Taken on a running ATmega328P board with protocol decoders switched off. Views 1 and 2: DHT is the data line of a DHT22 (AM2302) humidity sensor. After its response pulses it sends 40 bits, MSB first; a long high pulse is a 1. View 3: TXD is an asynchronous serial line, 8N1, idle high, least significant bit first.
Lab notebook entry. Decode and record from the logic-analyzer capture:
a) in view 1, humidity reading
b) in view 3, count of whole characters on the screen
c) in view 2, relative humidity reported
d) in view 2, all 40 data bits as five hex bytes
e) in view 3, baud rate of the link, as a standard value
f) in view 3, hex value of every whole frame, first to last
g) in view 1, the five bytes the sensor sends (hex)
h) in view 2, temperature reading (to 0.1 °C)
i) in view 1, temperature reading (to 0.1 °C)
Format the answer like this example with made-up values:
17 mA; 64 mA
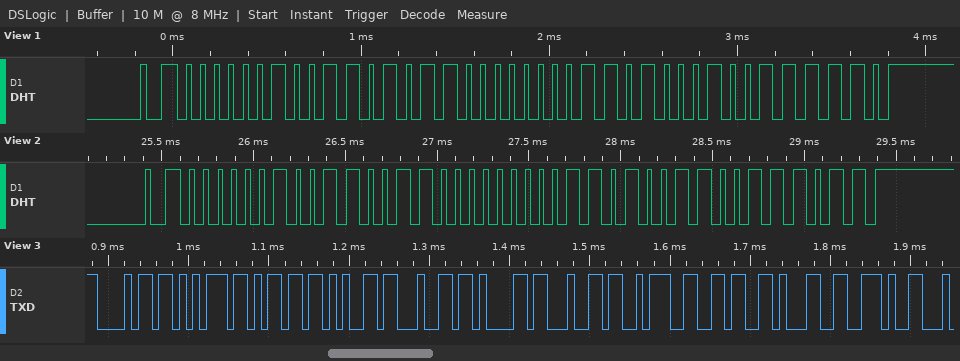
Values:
61.9 %; 11; 61.4 %; 02 66 00 D3 3B; 115200 baud; 68 75 6D 65 64 61 64 3A 36 31 2E; 02 6B 00 D1 3E; 21.1 °C; 20.9 °C
